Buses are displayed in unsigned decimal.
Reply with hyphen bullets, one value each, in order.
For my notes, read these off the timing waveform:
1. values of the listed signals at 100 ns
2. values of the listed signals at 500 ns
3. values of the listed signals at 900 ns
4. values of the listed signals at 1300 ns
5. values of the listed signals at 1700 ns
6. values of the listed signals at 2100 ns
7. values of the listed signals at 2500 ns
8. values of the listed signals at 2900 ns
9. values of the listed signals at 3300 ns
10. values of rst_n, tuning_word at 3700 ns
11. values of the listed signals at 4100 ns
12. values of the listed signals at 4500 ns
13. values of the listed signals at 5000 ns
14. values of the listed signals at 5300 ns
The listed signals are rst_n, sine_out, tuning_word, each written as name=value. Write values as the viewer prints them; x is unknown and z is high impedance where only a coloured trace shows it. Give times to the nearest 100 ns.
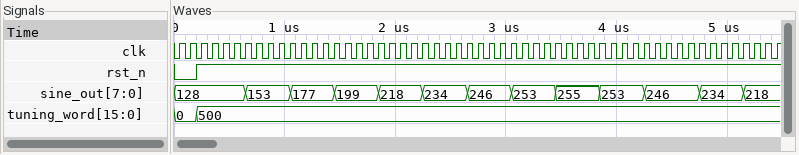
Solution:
- rst_n=0, sine_out=128, tuning_word=0
- rst_n=1, sine_out=128, tuning_word=500
- rst_n=1, sine_out=153, tuning_word=500
- rst_n=1, sine_out=177, tuning_word=500
- rst_n=1, sine_out=199, tuning_word=500
- rst_n=1, sine_out=218, tuning_word=500
- rst_n=1, sine_out=234, tuning_word=500
- rst_n=1, sine_out=246, tuning_word=500
- rst_n=1, sine_out=253, tuning_word=500
- rst_n=1, tuning_word=500
- rst_n=1, sine_out=253, tuning_word=500
- rst_n=1, sine_out=246, tuning_word=500
- rst_n=1, sine_out=234, tuning_word=500
- rst_n=1, sine_out=218, tuning_word=500
